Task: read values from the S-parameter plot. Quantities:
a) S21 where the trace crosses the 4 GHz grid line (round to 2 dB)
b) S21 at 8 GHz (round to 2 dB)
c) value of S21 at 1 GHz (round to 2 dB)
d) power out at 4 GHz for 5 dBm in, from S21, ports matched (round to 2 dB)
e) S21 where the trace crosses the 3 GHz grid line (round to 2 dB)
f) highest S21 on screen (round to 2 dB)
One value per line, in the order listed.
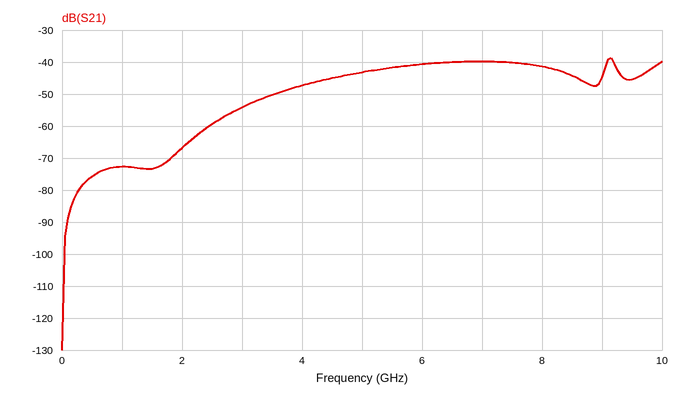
-48 dB
-42 dB
-72 dB
-42 dBm
-54 dB
-38 dB
